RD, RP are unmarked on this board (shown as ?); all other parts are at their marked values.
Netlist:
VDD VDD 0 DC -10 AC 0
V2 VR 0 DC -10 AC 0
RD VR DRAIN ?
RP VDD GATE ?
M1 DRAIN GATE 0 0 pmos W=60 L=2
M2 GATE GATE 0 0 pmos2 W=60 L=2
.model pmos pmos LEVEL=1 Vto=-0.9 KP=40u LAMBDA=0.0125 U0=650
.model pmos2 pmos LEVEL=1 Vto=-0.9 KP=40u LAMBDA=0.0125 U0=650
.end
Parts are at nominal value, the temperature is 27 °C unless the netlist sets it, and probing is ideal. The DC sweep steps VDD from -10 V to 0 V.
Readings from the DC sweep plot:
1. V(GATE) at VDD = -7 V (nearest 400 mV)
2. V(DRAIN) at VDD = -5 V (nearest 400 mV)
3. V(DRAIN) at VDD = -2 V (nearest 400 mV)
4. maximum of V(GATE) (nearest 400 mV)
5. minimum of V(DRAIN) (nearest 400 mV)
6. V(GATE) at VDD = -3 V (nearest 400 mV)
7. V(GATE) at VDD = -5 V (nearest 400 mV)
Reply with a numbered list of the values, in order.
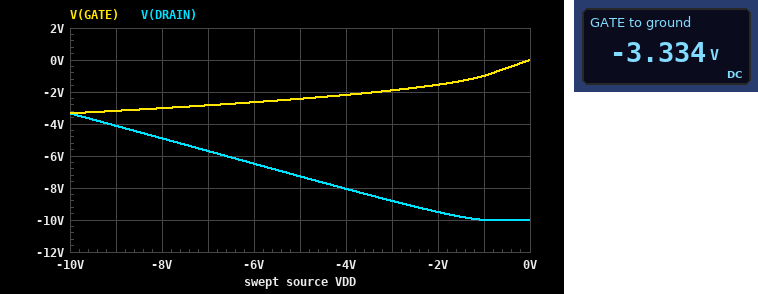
1. -2.8 V
2. -7.2 V
3. -9.6 V
4. 0 V
5. -10.0 V
6. -2.0 V
7. -2.4 V
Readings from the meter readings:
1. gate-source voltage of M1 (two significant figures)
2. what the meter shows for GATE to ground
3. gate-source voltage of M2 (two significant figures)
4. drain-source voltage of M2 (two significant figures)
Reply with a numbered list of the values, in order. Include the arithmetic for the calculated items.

1. -3.334 V = -3.3 V
2. -3.334 V
3. -3.334 V = -3.3 V
4. -3.334 V = -3.3 V
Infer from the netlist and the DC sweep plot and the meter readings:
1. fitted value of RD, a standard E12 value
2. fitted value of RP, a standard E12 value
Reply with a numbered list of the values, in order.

1. 1.8 kΩ
2. 1.8 kΩ
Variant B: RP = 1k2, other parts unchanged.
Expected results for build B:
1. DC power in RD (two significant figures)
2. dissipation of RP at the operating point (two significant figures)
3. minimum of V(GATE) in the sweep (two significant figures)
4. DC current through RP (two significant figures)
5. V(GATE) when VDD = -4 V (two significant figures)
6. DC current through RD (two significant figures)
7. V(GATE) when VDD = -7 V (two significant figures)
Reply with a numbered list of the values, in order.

1. 36 mW
2. 32 mW
3. -3.8 V
4. 5.2 mA
5. -2.4 V
6. 4.5 mA
7. -3.2 V
